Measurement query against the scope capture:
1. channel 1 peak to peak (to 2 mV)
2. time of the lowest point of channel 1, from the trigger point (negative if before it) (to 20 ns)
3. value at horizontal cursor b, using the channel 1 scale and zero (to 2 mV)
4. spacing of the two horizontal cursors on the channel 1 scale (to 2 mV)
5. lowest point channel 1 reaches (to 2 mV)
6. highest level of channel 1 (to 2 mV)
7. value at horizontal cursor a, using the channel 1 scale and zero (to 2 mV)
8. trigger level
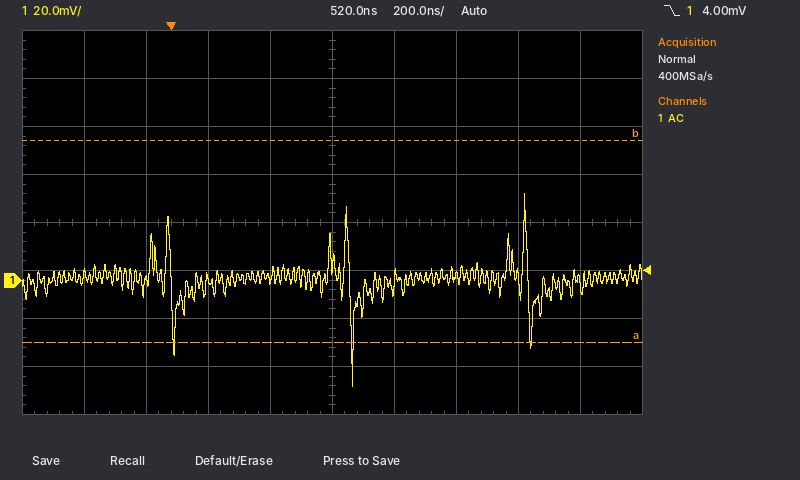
80 mV
+580 ns
58 mV
84 mV
-44 mV
36 mV
-26 mV
4.00 mV
